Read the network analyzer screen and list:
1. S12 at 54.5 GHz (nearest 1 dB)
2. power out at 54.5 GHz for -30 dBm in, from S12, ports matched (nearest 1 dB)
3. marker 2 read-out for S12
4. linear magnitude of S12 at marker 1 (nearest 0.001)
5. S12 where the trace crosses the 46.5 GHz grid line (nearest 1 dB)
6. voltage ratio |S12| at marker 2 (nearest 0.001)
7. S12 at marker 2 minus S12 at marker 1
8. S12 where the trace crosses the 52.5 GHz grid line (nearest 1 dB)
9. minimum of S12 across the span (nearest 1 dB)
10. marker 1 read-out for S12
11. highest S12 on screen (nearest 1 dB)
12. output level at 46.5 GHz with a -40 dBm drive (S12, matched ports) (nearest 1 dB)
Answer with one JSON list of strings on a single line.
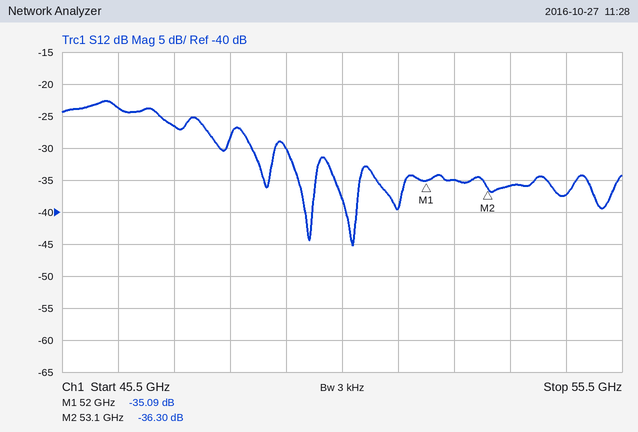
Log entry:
["-37 dB", "-67 dBm", "-36.30 dB", "0.018", "-24 dB", "0.015", "-1.21 dB", "-35 dB", "-45 dB", "-35.09 dB", "-23 dB", "-64 dBm"]
